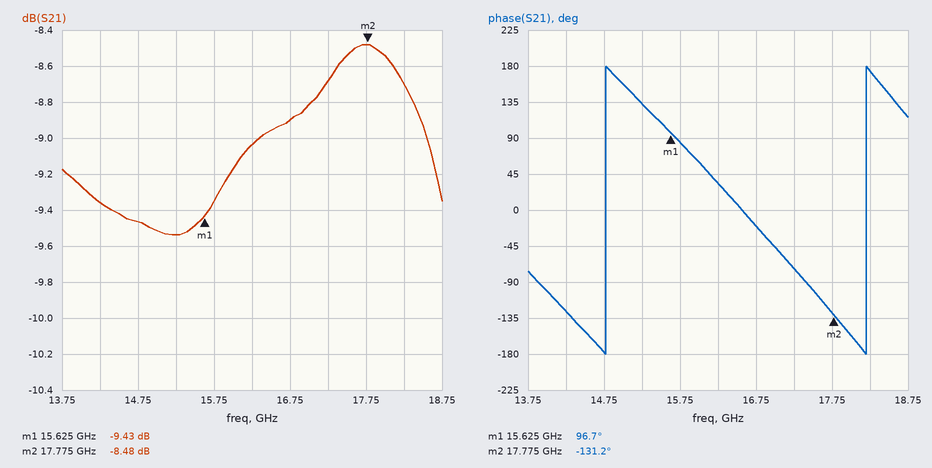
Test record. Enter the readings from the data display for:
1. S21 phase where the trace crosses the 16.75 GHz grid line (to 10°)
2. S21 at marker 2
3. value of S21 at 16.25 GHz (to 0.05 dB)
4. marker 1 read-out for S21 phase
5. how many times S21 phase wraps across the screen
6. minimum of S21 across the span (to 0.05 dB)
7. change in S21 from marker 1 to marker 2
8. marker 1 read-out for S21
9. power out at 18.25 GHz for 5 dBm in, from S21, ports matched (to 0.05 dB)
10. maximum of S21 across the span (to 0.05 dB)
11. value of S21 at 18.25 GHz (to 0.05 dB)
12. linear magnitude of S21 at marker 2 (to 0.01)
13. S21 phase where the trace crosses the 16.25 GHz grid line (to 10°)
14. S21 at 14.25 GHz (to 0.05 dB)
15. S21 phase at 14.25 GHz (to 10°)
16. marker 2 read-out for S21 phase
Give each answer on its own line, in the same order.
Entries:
-20°
-8.48 dB
-9.05 dB
96.7°
2
-9.55 dB
0.95 dB
-9.43 dB
-3.70 dBm
-8.50 dB
-8.70 dB
0.38
30°
-9.35 dB
-130°
-131.2°
